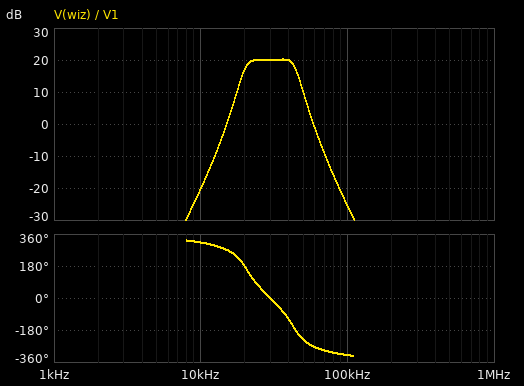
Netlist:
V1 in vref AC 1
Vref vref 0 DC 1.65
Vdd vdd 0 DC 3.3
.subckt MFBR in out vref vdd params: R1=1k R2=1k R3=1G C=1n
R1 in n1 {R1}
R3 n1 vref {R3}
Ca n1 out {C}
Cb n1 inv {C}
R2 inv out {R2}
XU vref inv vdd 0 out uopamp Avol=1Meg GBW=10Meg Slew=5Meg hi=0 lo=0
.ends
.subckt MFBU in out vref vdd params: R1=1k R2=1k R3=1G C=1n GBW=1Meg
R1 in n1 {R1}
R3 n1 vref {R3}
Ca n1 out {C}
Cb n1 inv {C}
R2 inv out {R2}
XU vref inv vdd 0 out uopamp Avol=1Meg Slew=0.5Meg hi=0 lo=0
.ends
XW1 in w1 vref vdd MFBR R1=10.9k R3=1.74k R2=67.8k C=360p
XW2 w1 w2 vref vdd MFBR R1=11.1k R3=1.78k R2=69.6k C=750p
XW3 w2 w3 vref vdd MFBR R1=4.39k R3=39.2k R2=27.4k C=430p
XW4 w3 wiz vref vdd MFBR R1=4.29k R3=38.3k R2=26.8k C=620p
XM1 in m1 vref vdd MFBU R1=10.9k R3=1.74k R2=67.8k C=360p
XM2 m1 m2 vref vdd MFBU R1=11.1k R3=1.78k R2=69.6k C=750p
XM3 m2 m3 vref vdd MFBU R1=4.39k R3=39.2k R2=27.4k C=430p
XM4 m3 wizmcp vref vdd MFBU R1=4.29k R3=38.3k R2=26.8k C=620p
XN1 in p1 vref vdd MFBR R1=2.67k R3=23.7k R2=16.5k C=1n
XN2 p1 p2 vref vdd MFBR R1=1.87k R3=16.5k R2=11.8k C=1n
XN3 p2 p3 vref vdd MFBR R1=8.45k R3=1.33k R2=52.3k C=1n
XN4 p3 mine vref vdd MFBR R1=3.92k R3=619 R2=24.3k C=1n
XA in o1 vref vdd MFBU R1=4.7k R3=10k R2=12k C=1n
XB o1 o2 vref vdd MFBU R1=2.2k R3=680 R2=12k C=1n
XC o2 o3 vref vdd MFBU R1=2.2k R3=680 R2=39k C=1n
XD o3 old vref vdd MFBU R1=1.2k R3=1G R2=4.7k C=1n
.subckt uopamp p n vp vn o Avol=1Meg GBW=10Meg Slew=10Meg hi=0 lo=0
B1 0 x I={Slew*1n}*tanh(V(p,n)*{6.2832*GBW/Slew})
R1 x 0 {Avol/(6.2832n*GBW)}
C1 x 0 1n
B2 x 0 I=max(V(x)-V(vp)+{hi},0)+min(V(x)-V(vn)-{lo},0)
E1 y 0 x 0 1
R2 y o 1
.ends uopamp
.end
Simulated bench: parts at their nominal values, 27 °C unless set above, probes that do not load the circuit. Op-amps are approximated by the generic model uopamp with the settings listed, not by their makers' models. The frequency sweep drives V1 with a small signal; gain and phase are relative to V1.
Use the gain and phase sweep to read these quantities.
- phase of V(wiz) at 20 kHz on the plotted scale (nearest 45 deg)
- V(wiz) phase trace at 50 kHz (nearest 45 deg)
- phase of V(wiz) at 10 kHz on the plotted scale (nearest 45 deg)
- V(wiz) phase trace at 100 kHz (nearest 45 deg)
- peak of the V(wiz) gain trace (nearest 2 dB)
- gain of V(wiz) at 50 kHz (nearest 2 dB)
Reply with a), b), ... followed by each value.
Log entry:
a) 180 deg
b) -225 deg
c) 315 deg
d) -315 deg
e) 20 dB
f) 10 dB
